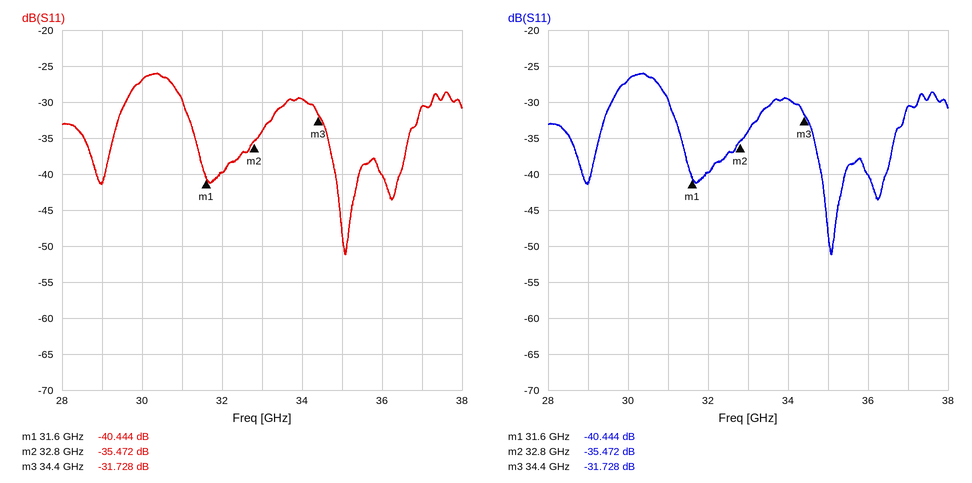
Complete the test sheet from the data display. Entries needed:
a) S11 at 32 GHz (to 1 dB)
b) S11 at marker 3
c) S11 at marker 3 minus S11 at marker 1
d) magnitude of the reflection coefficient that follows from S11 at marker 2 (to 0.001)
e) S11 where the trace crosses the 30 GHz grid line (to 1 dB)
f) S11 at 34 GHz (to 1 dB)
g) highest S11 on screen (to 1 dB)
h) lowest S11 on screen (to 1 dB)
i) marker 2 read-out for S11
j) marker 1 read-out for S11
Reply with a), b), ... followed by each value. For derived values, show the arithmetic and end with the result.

a) -40 dB
b) -31.728 dB
c) -31.728 − (-40.444) = 8.716 dB
d) 10^(-35.472/20) ≈ 0.017
e) -27 dB
f) -30 dB
g) -26 dB
h) -51 dB
i) -35.472 dB
j) -40.444 dB
